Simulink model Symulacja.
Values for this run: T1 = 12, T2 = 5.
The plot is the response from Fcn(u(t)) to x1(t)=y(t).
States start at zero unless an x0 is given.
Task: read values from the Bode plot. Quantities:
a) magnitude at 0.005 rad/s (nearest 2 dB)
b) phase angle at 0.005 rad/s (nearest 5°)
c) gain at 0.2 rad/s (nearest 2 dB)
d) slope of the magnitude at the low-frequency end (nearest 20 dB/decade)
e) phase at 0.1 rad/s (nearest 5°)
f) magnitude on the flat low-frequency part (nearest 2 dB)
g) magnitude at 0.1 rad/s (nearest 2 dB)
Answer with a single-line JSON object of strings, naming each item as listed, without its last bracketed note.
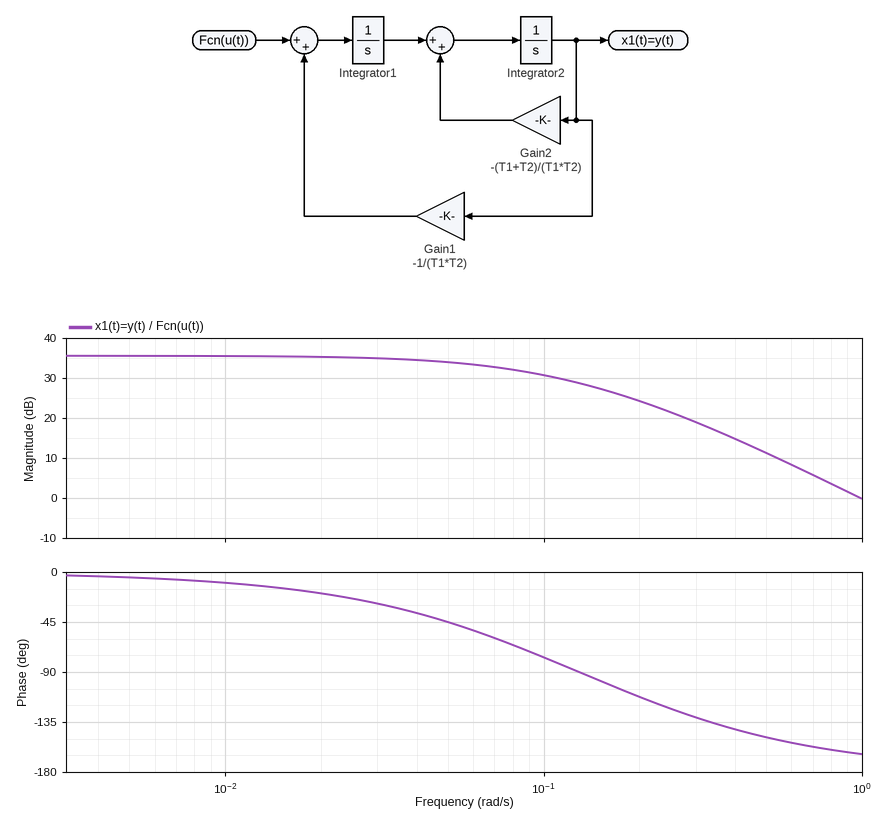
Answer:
{"magnitude at 0.005 rad/s": "36 dB", "phase angle at 0.005 rad/s": "-5°", "gain at 0.2 rad/s": "24 dB", "slope of the magnitude at the low-frequency end": "0 dB/decade", "phase at 0.1 rad/s": "-75°", "magnitude on the flat low-frequency part": "36 dB", "magnitude at 0.1 rad/s": "30 dB"}
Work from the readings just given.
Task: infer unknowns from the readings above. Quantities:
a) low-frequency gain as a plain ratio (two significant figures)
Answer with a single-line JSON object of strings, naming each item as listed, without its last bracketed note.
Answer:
{"low-frequency gain as a plain ratio": "63"}
